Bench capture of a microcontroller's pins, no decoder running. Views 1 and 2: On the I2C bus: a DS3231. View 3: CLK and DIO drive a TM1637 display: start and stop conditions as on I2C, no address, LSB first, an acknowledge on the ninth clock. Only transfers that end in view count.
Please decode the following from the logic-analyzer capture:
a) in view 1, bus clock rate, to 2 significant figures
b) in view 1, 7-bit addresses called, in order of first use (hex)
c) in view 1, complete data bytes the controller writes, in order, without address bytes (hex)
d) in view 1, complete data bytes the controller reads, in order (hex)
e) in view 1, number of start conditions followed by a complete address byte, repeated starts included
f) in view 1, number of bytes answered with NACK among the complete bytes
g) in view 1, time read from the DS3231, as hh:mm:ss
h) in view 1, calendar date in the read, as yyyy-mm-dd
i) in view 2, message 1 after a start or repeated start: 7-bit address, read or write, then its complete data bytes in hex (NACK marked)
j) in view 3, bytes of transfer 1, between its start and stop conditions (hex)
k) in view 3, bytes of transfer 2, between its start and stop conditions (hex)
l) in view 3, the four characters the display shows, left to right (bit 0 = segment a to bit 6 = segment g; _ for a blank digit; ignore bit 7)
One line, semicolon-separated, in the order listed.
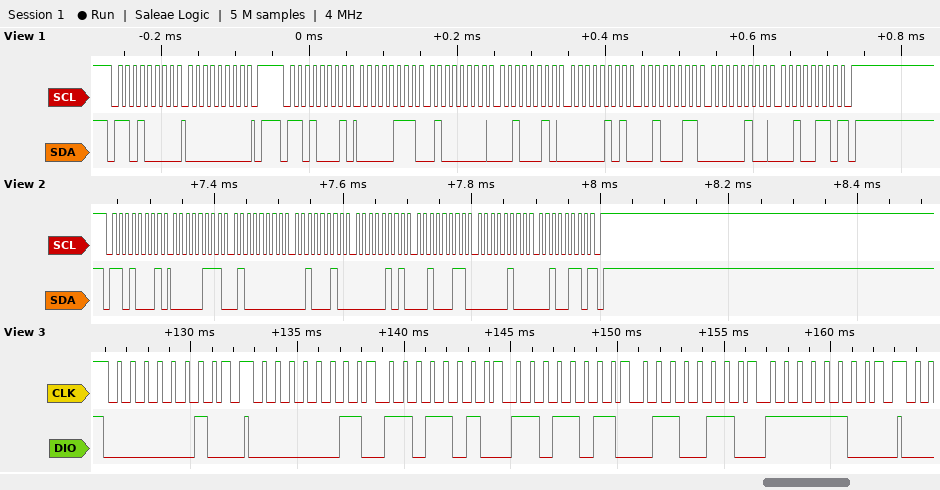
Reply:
100 kHz; 0x68; 00; 07 40 22 05 23 04 26; 2; 1; 22:40:07; 2026-04-23; 0x68 read: 07 40 22 05 23 04 26 NACK; 40; C0 5B DB 66 3F; 2240
